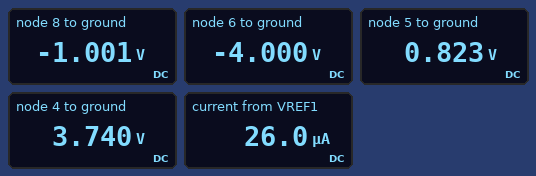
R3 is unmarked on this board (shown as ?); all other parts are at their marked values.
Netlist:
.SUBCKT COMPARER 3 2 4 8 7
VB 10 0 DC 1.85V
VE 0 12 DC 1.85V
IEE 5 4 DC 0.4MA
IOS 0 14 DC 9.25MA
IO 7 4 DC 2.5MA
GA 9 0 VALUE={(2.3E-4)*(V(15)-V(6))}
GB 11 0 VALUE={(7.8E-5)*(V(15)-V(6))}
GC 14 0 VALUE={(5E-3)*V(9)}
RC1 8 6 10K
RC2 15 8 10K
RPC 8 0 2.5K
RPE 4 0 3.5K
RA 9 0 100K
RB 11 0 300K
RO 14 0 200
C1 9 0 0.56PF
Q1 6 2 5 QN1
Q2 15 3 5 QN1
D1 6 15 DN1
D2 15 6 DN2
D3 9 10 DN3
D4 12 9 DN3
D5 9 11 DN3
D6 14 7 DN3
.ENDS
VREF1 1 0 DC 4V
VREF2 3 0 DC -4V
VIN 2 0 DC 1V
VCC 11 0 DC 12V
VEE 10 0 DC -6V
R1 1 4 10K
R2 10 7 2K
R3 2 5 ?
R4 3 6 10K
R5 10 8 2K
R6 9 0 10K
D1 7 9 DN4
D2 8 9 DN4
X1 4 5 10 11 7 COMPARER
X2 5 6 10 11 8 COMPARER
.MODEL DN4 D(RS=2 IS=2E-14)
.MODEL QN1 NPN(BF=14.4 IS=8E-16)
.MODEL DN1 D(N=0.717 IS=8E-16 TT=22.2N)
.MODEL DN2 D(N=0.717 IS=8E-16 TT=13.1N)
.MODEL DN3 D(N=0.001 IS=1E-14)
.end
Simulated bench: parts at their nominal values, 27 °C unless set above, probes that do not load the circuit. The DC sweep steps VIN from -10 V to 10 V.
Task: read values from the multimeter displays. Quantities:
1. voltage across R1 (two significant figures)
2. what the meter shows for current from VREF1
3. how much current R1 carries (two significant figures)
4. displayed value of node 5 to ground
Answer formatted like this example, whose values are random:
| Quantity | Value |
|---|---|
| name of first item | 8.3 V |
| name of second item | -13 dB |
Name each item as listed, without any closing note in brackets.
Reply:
| Quantity | Value |
|---|---|
| voltage across R1 | 260 mV |
| what the meter shows for current from VREF1 | 26.0 µA |
| how much current R1 carries | 26 µA |
| displayed value of node 5 to ground | 0.823 V |
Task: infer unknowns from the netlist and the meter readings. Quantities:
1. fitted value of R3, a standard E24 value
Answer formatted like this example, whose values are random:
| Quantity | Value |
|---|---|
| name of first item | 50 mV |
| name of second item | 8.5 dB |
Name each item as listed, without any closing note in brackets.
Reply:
| Quantity | Value |
|---|---|
| fitted value of R3, a standard E24 value | 6.8 kΩ |
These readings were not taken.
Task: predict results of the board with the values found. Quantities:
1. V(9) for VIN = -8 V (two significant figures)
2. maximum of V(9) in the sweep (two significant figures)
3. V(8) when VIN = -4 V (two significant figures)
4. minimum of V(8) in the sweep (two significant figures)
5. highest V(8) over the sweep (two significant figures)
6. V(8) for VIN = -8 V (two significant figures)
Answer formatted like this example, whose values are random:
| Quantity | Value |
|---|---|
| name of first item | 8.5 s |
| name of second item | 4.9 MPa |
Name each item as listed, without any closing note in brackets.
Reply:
| Quantity | Value |
|---|---|
| V(9) for VIN = -8 V | 1.7 V |
| maximum of V(9) in the sweep | 1.7 V |
| V(8) when VIN = -4 V | -1.0 V |
| minimum of V(8) in the sweep | -1.0 V |
| highest V(8) over the sweep | 2.3 V |
| V(8) for VIN = -8 V | 2.3 V |
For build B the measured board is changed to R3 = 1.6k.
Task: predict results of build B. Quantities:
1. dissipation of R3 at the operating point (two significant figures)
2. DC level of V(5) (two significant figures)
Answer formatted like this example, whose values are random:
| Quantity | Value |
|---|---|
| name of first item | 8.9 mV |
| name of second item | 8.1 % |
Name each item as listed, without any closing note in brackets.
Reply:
| Quantity | Value |
|---|---|
| dissipation of R3 at the operating point | 1.1 µW |
| DC level of V(5) | 960 mV |
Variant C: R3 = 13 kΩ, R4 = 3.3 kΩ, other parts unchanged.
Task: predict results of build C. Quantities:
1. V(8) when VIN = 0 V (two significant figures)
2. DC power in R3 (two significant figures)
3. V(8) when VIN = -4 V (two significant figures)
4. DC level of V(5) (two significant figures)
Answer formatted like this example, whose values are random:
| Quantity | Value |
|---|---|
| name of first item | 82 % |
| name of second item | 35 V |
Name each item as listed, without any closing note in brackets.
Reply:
| Quantity | Value |
|---|---|
| V(8) when VIN = 0 V | -1.0 V |
| DC power in R3 | 8.8 µW |
| V(8) when VIN = -4 V | 2.3 V |
| DC level of V(5) | 660 mV |
